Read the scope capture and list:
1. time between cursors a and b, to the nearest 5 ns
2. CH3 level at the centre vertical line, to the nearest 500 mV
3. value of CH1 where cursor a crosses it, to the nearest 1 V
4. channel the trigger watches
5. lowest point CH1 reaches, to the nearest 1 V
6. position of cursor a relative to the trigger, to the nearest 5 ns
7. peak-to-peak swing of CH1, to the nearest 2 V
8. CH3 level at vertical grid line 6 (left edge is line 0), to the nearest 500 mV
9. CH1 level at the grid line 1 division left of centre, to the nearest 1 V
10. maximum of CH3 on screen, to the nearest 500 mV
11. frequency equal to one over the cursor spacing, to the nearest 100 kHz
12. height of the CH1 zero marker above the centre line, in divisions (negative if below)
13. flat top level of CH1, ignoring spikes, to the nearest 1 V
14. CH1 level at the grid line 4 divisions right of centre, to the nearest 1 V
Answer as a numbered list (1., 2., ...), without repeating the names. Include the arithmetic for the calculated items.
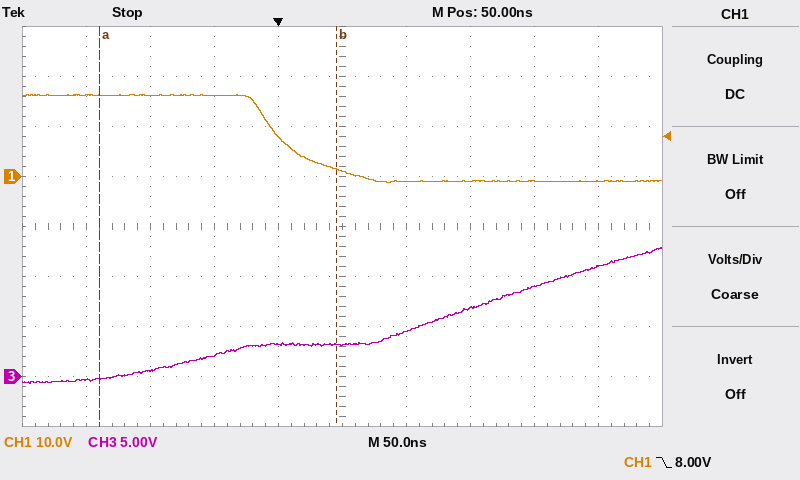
1. 185 ns
2. 3.0 V
3. 16 V
4. CH1
5. -1 V
6. -140 ns
7. 18 V
8. 4.5 V
9. 8 V
10. 13.0 V
11. 1 / 185 ns ≈ 5.4 MHz
12. +1.0 div
13. 16 V
14. -1 V
